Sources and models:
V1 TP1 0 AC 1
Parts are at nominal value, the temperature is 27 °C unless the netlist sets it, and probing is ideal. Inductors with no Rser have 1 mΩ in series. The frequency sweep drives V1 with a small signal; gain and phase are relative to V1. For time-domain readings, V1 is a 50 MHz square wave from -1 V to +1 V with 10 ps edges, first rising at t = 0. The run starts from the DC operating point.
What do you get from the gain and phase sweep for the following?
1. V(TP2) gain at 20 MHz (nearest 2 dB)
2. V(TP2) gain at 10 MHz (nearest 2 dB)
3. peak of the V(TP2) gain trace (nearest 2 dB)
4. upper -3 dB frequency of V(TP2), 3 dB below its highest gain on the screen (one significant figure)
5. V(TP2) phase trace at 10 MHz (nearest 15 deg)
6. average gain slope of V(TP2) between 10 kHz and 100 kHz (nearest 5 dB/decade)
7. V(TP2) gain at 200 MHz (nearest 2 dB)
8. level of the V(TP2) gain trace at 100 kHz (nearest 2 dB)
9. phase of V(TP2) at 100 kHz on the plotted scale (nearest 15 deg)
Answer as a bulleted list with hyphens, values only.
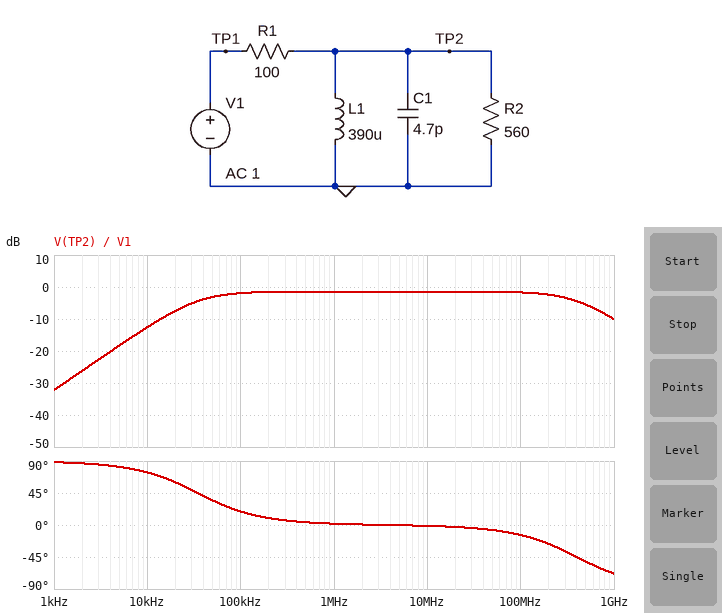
- -2 dB
- -2 dB
- -2 dB
- 400 MHz
- 0 deg
- 10 dB/decade
- -2 dB
- -2 dB
- 15 deg
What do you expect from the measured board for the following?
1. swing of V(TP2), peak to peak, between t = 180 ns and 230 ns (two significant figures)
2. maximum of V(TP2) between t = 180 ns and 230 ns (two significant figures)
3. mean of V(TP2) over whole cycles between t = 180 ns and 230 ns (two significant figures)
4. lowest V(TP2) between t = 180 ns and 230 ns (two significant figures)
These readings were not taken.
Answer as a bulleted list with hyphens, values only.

- 1.7 V
- 1.7 V
- 810 mV
- -40 mV
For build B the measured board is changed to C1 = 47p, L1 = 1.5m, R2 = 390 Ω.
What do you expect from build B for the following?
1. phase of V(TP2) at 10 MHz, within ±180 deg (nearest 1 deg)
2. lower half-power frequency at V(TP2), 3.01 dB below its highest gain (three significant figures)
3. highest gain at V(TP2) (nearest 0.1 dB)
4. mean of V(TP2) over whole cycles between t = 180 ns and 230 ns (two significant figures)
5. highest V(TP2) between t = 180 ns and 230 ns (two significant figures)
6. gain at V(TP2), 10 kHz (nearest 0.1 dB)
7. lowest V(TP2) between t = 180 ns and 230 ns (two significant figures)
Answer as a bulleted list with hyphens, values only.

- -13 deg
- 8.44 kHz
- -2.0 dB
- 790 mV
- 1.5 V
- -4.3 dB
- 94 mV
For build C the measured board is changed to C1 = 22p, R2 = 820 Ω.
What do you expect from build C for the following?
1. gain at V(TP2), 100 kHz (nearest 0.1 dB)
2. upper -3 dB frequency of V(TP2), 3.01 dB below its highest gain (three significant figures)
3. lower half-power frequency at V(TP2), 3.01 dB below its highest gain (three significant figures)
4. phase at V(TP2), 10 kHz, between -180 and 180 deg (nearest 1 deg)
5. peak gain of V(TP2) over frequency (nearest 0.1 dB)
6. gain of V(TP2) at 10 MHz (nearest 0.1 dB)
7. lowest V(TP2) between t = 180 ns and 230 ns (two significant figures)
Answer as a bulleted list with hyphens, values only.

- -1.5 dB
- 81.2 MHz
- 36.4 kHz
- 75 deg
- -1.0 dB
- -1.1 dB
- -33 mV
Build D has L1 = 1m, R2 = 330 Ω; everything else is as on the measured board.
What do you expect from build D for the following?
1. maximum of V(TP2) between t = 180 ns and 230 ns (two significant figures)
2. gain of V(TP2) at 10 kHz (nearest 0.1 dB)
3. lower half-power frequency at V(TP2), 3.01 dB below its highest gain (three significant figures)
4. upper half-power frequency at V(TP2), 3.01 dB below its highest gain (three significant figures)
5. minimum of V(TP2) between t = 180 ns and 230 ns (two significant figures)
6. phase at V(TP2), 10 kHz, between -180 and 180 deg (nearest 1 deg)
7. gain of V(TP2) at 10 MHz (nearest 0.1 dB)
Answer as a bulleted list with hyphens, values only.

- 1.5 V
- -6.3 dB
- 12.2 kHz
- 441 MHz
- -13 mV
- 51 deg
- -2.3 dB
